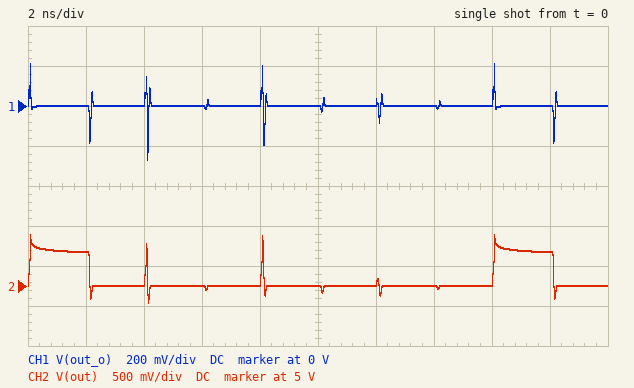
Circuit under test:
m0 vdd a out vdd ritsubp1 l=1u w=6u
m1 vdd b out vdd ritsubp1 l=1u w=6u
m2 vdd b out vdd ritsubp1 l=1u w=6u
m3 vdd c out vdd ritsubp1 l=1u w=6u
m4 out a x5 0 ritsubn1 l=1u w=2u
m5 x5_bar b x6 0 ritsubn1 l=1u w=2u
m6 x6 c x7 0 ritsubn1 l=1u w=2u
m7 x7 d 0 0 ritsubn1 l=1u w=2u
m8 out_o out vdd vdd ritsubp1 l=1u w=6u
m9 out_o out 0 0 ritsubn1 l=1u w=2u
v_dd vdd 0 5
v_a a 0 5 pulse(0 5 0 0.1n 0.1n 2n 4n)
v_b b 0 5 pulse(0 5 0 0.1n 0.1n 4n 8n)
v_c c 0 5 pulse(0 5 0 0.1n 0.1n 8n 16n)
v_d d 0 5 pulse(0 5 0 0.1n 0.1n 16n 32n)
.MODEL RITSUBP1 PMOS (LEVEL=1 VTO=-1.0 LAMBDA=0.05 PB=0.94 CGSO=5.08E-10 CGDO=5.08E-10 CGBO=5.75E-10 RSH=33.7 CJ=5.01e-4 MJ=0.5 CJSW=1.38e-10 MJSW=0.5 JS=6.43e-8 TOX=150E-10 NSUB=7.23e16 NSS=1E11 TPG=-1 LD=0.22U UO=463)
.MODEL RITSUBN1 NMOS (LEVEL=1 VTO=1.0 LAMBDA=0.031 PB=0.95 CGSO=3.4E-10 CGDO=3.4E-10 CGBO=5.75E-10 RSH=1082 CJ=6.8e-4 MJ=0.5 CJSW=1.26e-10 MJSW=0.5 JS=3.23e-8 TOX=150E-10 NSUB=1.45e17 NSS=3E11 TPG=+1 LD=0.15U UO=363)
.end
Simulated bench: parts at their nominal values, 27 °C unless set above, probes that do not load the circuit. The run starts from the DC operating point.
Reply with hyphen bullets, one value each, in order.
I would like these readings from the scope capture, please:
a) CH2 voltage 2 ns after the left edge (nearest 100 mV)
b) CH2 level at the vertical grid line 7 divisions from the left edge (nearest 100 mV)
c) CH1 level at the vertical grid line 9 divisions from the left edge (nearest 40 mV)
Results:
- 5.4 V
- 5.0 V
- 0 V
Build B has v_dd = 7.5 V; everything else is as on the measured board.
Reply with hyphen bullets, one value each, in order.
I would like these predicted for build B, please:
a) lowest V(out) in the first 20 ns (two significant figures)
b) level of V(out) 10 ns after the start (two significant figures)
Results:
- 7.4 V
- 7.5 V
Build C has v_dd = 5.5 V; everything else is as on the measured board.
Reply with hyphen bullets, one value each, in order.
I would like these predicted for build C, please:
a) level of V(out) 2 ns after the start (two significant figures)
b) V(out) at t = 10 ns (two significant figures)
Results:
- 5.9 V
- 5.5 V
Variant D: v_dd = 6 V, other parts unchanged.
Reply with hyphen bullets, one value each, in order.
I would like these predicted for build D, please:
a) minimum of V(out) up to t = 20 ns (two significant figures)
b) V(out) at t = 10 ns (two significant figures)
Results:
- 5.8 V
- 6.0 V
